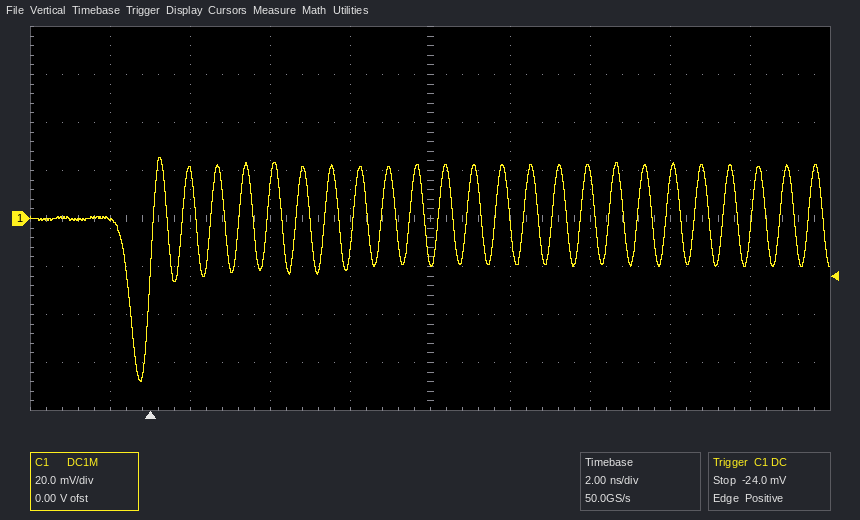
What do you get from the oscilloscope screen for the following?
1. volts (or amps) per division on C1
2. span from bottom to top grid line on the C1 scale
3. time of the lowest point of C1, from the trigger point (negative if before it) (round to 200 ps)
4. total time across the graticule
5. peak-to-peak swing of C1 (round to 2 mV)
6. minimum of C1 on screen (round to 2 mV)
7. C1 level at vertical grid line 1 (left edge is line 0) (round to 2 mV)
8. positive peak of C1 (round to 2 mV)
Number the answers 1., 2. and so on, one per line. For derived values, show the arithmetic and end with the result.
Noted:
1. 20 mV
2. 160 mV
3. -200 ps
4. 20 ns
5. 26 mV − (-68 mV) = 94 mV
6. -68 mV
7. 0 mV
8. 26 mV
